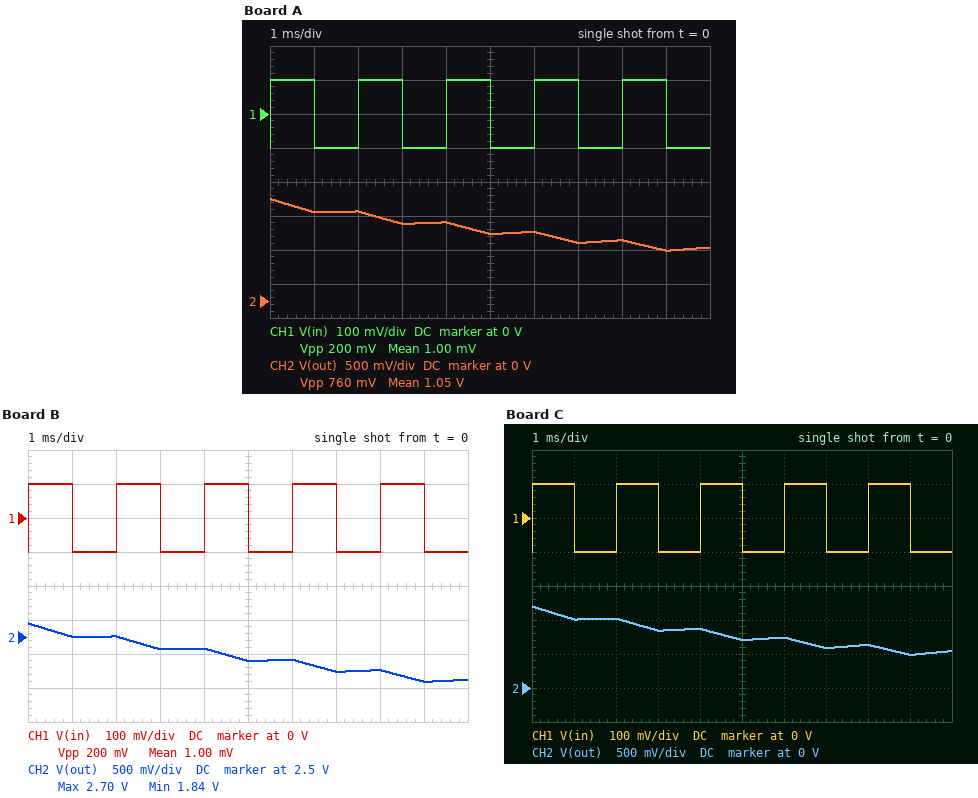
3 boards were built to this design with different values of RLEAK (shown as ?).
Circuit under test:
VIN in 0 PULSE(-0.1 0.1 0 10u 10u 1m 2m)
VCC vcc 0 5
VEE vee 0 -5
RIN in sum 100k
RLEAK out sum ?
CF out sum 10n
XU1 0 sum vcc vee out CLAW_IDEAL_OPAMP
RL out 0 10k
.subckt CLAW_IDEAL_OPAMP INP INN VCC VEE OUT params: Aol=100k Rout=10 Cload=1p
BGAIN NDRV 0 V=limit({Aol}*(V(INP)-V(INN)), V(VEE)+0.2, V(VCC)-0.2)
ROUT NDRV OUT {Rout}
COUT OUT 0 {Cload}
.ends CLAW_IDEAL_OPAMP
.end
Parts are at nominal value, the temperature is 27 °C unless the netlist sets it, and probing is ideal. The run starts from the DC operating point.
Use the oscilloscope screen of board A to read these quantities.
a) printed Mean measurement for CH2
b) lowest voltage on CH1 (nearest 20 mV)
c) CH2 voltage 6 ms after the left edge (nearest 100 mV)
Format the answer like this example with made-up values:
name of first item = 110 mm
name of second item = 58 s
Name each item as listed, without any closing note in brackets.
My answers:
printed Mean measurement for CH2 = 1.05 V
lowest voltage on CH1 = -100 mV
CH2 voltage 6 ms after the left edge = 1.0 V
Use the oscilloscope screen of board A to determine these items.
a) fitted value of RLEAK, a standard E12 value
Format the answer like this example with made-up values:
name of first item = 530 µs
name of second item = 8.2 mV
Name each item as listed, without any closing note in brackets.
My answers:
fitted value of RLEAK, a standard E12 value = 1.5 MΩ
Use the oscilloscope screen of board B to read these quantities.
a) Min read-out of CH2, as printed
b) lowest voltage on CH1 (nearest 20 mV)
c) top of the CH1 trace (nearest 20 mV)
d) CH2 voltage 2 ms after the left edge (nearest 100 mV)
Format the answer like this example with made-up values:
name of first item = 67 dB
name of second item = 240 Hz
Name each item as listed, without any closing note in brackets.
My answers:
Min read-out of CH2, as printed = 1.84 V
lowest voltage on CH1 = -100 mV
top of the CH1 trace = 100 mV
CH2 voltage 2 ms after the left edge = 2.5 V
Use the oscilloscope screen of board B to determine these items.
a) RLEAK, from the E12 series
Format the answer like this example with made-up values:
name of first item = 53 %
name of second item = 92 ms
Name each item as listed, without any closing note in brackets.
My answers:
RLEAK, from the E12 series = 2.7 MΩ
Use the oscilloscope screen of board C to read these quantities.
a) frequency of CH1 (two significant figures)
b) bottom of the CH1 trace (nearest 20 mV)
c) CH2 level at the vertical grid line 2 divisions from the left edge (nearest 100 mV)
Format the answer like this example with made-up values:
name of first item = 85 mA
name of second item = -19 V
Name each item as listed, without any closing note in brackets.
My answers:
frequency of CH1 = 500 Hz
bottom of the CH1 trace = -100 mV
CH2 level at the vertical grid line 2 divisions from the left edge = 1.0 V
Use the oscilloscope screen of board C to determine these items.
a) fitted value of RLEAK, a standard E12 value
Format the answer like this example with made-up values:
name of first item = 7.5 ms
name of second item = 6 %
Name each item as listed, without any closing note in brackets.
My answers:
fitted value of RLEAK, a standard E12 value = 1.2 MΩ
